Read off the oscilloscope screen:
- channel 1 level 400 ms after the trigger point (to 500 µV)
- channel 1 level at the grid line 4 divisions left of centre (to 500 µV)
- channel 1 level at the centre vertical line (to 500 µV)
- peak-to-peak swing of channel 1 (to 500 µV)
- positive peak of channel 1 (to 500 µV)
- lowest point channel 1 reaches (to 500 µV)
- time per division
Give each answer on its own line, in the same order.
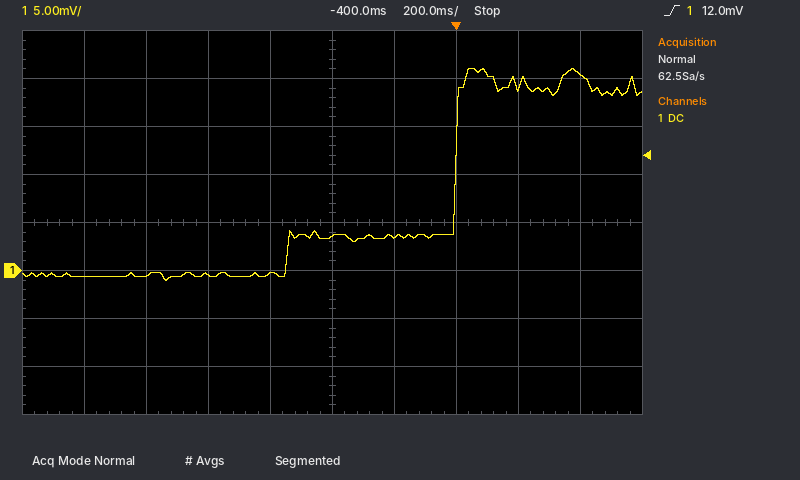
20.5 mV
-500 µV
3.5 mV
22.0 mV
21.0 mV
-1.0 mV
200 ms
